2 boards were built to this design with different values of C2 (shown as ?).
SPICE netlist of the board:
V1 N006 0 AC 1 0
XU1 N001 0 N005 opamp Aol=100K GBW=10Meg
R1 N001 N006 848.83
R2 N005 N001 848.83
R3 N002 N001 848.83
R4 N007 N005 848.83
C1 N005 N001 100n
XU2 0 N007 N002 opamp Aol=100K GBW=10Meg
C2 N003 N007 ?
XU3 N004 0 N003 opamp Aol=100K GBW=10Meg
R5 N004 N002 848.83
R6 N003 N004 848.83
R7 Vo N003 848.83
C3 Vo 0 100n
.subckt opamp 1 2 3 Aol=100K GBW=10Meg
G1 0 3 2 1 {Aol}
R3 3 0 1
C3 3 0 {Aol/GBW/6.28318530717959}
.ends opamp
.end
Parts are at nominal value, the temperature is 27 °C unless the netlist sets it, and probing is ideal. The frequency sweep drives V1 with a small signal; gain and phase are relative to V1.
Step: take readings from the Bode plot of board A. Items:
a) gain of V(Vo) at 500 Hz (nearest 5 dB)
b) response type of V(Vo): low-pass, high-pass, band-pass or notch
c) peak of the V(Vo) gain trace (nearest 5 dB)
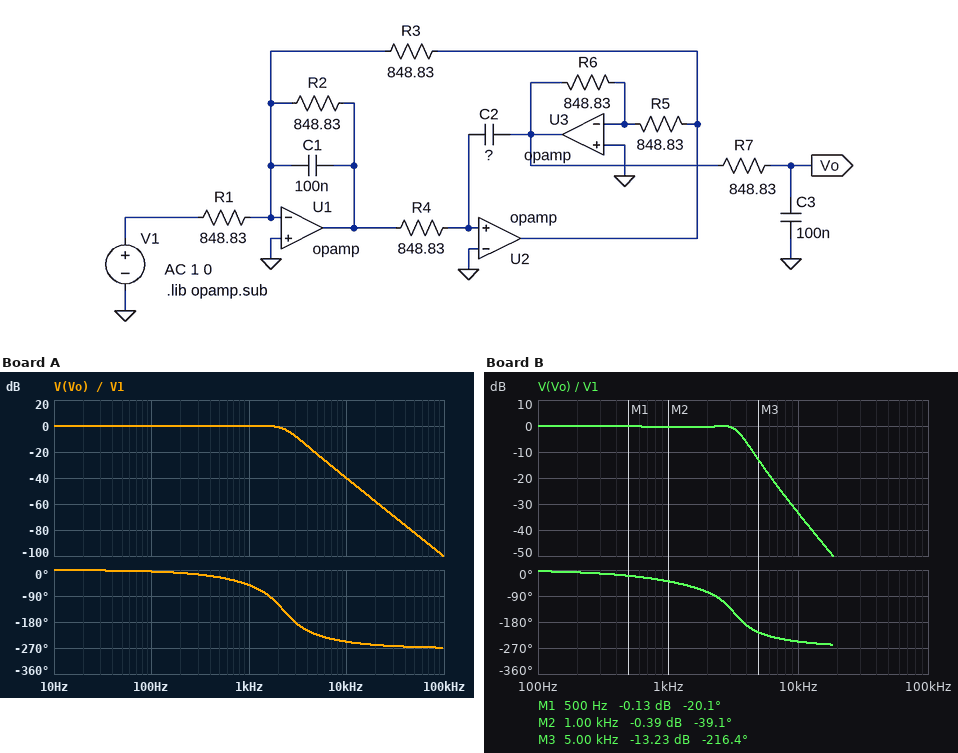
0 dB
low-pass
0 dB
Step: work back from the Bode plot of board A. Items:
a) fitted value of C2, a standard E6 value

68 nF
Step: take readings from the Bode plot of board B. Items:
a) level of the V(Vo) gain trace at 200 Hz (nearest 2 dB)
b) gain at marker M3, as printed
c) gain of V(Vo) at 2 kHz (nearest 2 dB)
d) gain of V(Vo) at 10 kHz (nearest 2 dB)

0 dB
-13.23 dB
0 dB
-34 dB
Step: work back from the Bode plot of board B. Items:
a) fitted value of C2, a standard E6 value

33 nF
